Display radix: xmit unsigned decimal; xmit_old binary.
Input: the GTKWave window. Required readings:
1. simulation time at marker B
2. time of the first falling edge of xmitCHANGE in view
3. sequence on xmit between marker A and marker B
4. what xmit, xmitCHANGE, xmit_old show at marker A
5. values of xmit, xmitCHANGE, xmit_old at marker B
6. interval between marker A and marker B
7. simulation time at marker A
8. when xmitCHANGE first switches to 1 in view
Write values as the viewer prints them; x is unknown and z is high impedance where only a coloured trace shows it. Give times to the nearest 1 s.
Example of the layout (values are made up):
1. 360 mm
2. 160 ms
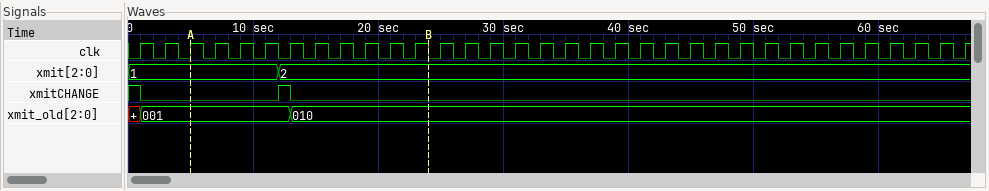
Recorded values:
1. 24 s
2. 1 s
3. 1, 2
4. xmit=1, xmitCHANGE=0, xmit_old=001
5. xmit=2, xmitCHANGE=0, xmit_old=010
6. 19 s
7. 5 s
8. 12 s
